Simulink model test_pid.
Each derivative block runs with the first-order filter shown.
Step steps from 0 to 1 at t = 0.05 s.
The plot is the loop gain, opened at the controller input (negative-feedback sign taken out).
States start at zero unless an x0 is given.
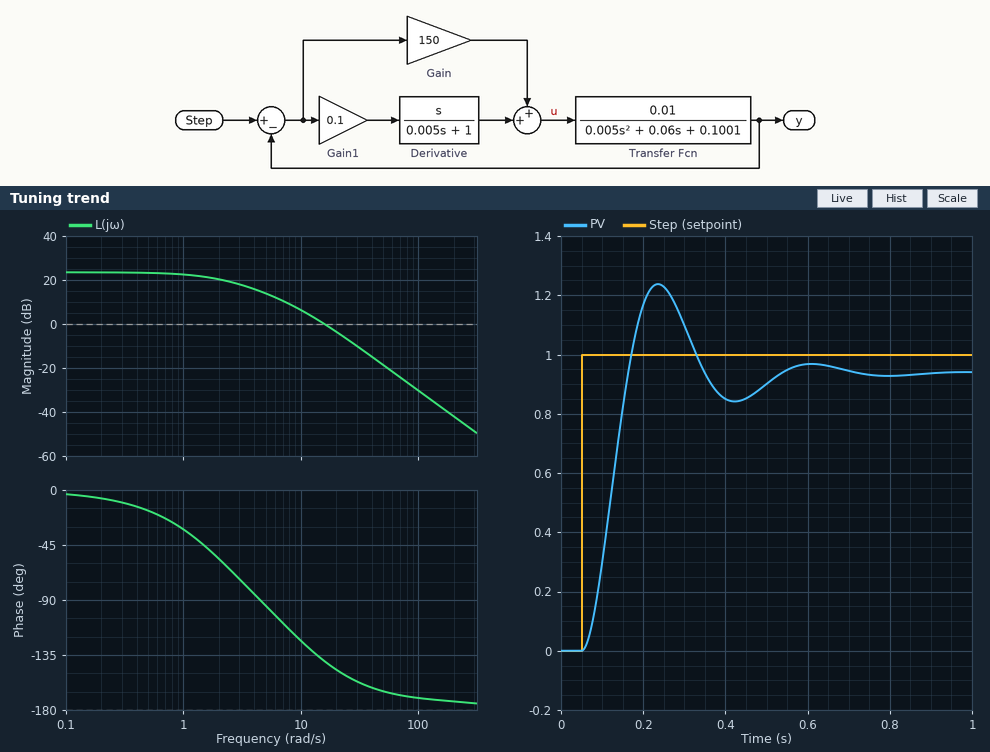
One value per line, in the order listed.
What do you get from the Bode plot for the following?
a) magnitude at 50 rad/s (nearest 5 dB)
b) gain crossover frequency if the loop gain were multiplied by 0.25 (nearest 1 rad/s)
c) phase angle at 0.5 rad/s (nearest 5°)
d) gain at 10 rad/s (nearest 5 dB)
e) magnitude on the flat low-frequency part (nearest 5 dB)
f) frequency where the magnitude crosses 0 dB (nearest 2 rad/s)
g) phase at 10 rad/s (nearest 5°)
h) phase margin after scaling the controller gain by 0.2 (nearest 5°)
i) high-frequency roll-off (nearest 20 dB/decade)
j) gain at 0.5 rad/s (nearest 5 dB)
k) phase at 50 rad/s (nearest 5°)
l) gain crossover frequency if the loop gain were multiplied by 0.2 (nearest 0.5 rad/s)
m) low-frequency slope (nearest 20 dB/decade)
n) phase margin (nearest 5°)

-20 dB
6 rad/s
-15°
5 dB
25 dB
16 rad/s
-125°
85°
-40 dB/decade
25 dB
-165°
5.0 rad/s
0 dB/decade
40°
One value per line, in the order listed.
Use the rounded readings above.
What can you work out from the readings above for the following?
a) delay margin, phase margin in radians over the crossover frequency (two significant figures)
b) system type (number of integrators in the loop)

0.044 s
0
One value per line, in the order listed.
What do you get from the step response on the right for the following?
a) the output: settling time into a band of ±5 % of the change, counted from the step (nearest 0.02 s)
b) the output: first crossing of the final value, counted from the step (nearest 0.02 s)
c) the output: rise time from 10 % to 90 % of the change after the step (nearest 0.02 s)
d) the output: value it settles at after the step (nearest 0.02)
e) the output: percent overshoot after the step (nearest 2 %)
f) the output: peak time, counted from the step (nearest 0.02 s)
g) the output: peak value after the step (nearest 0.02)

0.44 s
0.12 s
0.08 s
0.94
32 %
0.18 s
1.24
